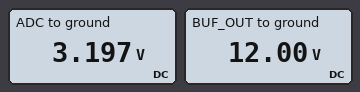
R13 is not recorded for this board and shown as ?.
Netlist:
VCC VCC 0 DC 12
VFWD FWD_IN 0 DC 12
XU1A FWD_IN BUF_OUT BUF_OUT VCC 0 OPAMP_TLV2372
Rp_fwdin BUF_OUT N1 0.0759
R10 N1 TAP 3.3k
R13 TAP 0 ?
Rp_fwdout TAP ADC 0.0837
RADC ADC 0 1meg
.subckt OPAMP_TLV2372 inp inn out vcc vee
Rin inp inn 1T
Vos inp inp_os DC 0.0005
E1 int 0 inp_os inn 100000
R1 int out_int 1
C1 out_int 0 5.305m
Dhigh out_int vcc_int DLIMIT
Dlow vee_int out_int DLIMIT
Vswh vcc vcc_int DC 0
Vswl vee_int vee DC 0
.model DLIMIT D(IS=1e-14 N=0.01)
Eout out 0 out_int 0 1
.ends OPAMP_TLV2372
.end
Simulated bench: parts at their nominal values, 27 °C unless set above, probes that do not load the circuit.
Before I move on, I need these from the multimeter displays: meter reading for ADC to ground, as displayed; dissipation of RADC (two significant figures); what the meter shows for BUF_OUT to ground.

3.197 V
10 µW
12.00 V
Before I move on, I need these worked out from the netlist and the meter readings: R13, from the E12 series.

1.2 kΩ
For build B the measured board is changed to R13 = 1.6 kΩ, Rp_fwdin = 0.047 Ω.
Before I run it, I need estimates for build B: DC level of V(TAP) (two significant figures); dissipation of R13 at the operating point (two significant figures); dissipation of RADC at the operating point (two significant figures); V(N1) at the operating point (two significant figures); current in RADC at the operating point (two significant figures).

3.9 V
9.6 mW
15 µW
12 V
3.9 µA
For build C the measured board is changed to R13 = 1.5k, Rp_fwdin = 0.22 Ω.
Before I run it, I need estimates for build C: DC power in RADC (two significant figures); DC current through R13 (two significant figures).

14 µW
2.5 mA
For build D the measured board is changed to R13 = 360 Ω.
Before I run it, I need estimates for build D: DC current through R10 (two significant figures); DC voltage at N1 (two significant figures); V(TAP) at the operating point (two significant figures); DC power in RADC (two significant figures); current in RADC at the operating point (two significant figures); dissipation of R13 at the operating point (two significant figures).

3.3 mA
12 V
1.2 V
1.4 µW
1.2 µA
3.9 mW
